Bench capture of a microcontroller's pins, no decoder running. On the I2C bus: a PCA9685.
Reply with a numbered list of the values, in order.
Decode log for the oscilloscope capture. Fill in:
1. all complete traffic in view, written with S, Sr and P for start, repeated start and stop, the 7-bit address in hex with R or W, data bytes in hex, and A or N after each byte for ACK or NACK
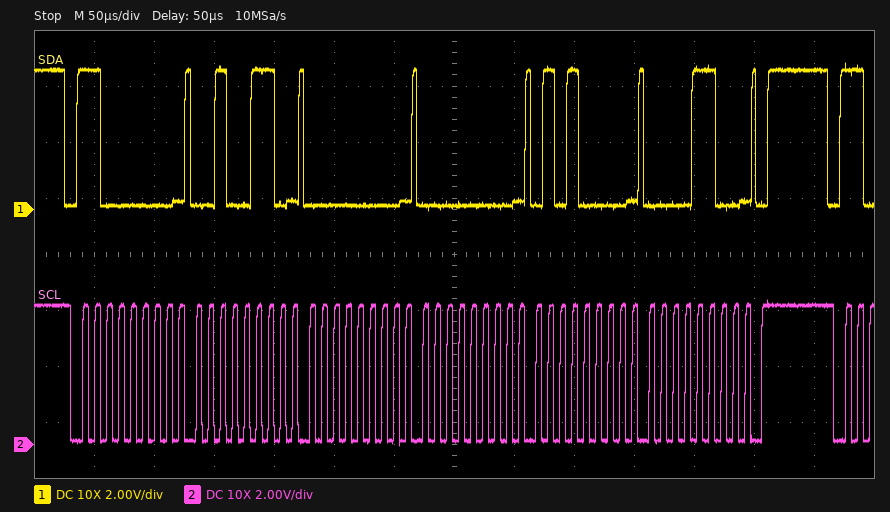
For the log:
1. S 60W A 26 A 00 A 00 A 50 A 0C A P
